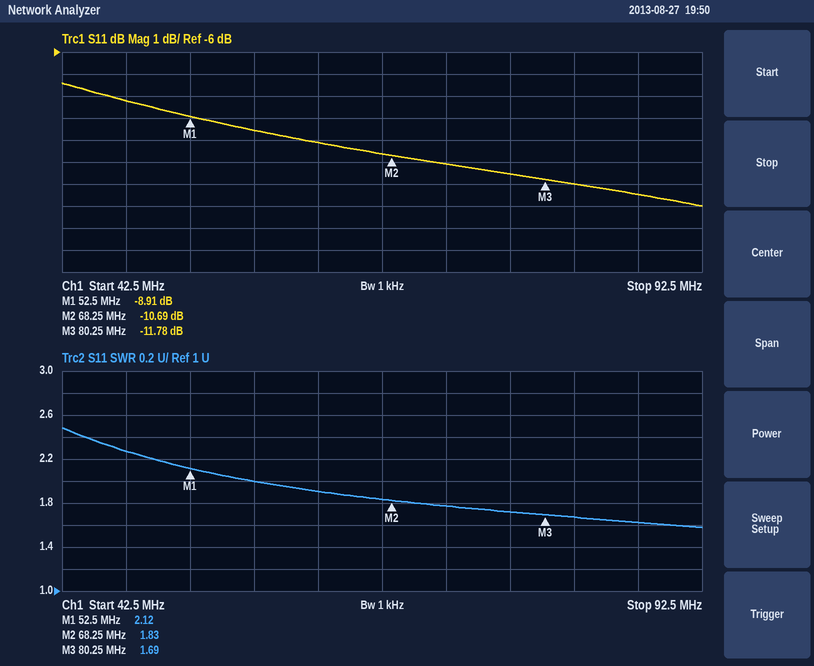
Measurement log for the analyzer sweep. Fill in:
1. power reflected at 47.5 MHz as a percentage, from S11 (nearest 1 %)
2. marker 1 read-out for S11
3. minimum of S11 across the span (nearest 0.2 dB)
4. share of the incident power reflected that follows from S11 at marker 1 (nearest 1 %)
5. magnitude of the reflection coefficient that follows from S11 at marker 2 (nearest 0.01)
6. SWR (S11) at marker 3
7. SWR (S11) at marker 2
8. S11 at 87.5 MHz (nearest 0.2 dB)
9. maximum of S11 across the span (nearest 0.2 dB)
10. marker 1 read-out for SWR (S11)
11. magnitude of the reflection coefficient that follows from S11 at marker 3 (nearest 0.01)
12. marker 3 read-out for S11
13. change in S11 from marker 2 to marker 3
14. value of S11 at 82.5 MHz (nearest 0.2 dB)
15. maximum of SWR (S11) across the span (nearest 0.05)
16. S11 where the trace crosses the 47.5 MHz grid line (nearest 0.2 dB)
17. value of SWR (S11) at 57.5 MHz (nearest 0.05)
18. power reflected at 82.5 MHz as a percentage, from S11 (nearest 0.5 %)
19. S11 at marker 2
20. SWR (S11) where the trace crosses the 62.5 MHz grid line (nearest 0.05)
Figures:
15 %
-8.91 dB
-13.0 dB
13 %
0.29
1.69
1.83
-12.4 dB
-7.4 dB
2.12
0.26
-11.78 dB
-1.09 dB
-12.0 dB
2.50
-8.2 dB
2.00
6.5 %
-10.69 dB
1.90
